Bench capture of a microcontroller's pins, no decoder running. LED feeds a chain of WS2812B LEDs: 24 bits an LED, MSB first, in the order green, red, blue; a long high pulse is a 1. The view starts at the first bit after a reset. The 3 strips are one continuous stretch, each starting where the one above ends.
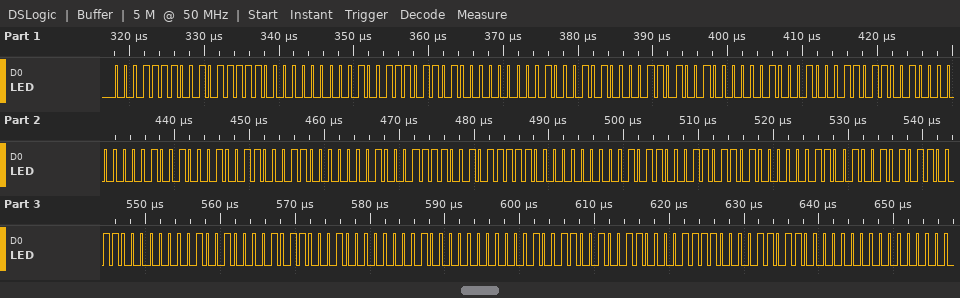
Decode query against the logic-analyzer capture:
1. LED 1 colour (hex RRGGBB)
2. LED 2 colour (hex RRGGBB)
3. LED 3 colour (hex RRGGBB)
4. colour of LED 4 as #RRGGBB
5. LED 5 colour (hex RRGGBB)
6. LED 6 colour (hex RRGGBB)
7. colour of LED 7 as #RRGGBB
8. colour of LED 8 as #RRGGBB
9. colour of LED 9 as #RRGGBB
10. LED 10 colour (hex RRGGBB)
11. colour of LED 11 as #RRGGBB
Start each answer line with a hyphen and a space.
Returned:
- #5F1E00
- #682702
- #692802
- #642301
- #632201
- #5F1E00
- #6D2C03
- #662501
- #622101
- #130026
- #1B1E00
